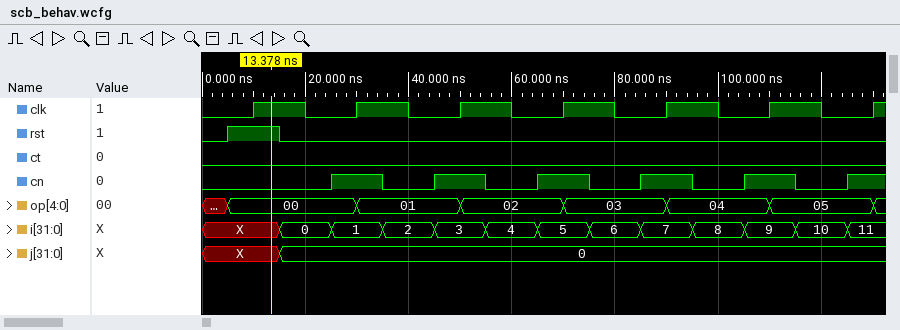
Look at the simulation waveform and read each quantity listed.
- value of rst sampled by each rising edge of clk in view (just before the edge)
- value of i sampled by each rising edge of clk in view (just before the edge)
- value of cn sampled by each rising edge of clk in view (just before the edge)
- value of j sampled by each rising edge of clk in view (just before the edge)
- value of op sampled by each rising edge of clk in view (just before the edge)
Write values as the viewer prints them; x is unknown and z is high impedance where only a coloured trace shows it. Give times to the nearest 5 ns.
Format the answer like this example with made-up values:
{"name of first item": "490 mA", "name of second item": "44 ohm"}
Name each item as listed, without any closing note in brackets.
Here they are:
{"value of rst sampled by each rising edge of clk in view": "1 0 0 0 0 0 0", "value of i sampled by each rising edge of clk in view": "X, 1, 3, 5, 7, 9, 11", "value of cn sampled by each rising edge of clk in view": "0 1 1 1 1 1 1", "value of j sampled by each rising edge of clk in view": "X, 0, 0, 0, 0, 0, 0", "value of op sampled by each rising edge of clk in view": "00, 00, 01, 02, 03, 04, 05"}
